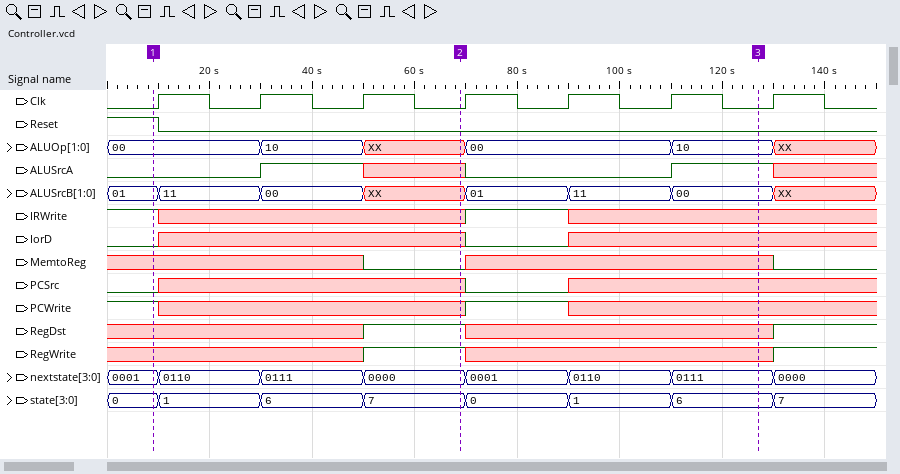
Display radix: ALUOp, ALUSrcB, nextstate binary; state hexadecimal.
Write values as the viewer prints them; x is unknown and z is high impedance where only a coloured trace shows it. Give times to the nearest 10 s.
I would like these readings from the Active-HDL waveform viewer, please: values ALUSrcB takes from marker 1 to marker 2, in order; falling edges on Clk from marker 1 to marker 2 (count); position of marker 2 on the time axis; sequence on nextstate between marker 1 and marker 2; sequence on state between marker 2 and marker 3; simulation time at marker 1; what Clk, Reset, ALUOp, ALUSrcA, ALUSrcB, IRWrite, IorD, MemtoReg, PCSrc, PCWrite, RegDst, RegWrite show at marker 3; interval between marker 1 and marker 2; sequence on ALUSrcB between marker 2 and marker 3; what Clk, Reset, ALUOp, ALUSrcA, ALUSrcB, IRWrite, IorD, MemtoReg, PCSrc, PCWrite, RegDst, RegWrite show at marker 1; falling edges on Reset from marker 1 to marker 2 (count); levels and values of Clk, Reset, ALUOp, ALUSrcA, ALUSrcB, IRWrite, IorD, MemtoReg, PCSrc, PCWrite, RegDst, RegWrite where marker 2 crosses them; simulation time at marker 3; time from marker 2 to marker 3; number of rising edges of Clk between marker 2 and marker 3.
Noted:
01, 11, 00, XX
3
70 s
0001, 0110, 0111, 0000
7, 0, 1, 6
10 s
Clk=0, Reset=0, ALUOp=10, ALUSrcA=1, ALUSrcB=00, IRWrite=x, IorD=x, MemtoReg=x, PCSrc=x, PCWrite=x, RegDst=x, RegWrite=x
60 s
XX, 01, 11, 00
Clk=0, Reset=1, ALUOp=00, ALUSrcA=0, ALUSrcB=01, IRWrite=1, IorD=0, MemtoReg=x, PCSrc=0, PCWrite=1, RegDst=x, RegWrite=x
1
Clk=0, Reset=0, ALUOp=XX, ALUSrcA=x, ALUSrcB=XX, IRWrite=x, IorD=x, MemtoReg=0, PCSrc=x, PCWrite=x, RegDst=1, RegWrite=1
130 s
60 s
3
